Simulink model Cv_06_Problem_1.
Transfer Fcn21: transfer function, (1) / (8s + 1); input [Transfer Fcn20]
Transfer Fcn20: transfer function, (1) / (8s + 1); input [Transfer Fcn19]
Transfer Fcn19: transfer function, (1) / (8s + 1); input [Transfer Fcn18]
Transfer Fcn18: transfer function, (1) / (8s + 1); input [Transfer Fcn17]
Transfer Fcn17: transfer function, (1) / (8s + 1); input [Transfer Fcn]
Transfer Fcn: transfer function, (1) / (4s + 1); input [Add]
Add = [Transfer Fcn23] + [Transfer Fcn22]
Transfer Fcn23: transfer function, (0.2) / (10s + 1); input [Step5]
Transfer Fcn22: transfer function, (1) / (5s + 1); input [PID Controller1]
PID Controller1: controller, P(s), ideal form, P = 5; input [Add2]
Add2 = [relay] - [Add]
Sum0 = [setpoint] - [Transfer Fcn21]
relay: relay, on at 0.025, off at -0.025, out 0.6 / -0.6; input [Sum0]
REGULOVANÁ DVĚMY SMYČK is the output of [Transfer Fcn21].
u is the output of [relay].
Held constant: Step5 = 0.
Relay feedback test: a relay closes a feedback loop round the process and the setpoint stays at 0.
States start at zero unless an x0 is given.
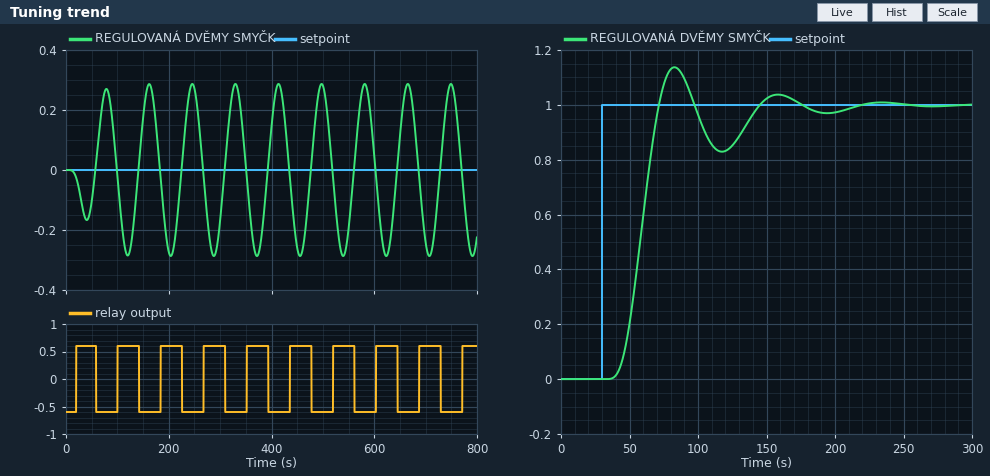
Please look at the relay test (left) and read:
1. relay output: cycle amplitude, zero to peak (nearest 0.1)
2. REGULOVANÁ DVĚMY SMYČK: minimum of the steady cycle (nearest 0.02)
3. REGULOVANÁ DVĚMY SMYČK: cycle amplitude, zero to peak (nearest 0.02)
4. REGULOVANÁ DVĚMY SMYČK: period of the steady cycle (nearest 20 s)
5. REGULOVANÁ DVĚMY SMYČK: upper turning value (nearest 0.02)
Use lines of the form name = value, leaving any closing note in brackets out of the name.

relay output: cycle amplitude, zero to peak = 0.6
REGULOVANÁ DVĚMY SMYČK: minimum of the steady cycle = -0.28
REGULOVANÁ DVĚMY SMYČK: cycle amplitude, zero to peak = 0.28
REGULOVANÁ DVĚMY SMYČK: period of the steady cycle = 80 s
REGULOVANÁ DVĚMY SMYČK: upper turning value = 0.28
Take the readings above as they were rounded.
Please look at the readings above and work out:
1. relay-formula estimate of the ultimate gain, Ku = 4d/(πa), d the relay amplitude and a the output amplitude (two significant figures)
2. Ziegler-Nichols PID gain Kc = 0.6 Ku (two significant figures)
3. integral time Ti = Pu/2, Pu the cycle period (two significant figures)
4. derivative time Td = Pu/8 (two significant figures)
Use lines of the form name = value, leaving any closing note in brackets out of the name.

relay-formula estimate of the ultimate gain, Ku = 4d/(πa), d the relay amplitude and a the output amplitude = 2.7
Ziegler-Nichols PID gain Kc = 0.6 Ku = 1.6
integral time Ti = Pu/2, Pu the cycle period = 40 s
derivative time Td = Pu/8 = 10 s
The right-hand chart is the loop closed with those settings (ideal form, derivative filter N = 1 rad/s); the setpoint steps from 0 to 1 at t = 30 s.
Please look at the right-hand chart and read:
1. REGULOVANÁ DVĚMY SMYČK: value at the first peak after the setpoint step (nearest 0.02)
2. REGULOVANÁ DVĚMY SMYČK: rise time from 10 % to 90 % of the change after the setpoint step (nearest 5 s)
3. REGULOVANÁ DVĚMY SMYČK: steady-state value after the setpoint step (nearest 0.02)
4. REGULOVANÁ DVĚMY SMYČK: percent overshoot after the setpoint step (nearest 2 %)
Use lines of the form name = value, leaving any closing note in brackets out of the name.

REGULOVANÁ DVĚMY SMYČK: value at the first peak after the setpoint step = 1.14
REGULOVANÁ DVĚMY SMYČK: rise time from 10 % to 90 % of the change after the setpoint step = 20 s
REGULOVANÁ DVĚMY SMYČK: steady-state value after the setpoint step = 1.00
REGULOVANÁ DVĚMY SMYČK: percent overshoot after the setpoint step = 14 %
